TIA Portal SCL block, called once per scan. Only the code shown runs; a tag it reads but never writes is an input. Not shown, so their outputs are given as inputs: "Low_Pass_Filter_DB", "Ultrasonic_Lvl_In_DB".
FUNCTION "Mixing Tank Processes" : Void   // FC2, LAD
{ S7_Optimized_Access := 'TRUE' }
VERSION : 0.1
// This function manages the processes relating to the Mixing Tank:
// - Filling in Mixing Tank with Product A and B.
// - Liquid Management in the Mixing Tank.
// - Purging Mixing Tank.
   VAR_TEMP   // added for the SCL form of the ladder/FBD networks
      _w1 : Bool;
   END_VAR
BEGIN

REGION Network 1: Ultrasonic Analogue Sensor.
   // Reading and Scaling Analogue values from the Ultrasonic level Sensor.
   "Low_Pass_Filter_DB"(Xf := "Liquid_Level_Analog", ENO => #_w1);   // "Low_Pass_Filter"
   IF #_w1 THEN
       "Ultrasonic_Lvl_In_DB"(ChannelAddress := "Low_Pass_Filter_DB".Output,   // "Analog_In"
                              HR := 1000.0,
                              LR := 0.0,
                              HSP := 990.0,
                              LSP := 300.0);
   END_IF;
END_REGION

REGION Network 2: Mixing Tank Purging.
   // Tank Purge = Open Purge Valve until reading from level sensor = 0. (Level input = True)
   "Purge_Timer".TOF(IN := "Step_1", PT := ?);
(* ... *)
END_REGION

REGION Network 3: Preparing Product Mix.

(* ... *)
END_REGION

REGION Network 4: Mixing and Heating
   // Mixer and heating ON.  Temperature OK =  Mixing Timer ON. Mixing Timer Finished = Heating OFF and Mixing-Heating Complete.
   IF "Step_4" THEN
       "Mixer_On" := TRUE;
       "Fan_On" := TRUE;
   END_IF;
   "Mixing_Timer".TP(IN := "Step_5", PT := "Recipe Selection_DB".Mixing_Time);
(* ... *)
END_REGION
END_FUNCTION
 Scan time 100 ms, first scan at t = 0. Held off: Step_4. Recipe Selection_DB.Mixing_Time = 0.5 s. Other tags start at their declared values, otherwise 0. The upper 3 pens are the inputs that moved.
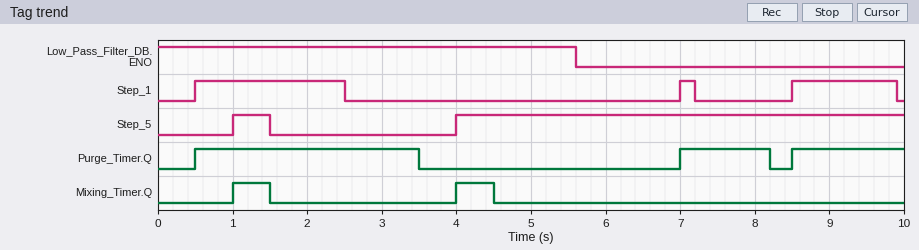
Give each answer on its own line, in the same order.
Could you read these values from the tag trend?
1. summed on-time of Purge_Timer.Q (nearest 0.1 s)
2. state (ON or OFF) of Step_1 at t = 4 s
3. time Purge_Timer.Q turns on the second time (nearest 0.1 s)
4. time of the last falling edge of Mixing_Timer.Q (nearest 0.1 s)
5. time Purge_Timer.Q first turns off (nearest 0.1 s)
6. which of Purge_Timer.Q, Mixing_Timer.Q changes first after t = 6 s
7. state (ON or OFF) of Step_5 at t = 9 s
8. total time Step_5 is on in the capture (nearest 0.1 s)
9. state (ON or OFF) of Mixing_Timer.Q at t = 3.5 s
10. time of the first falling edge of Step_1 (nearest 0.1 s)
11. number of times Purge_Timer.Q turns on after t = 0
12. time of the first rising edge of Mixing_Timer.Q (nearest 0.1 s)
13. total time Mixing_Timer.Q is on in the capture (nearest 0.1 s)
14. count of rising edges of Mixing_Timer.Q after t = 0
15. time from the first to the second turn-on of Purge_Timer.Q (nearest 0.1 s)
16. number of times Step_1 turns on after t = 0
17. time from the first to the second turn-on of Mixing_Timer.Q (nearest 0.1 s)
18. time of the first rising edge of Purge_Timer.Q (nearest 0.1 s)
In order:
5.7 s
OFF
7.0 s
4.5 s
3.5 s
Purge_Timer.Q
ON
6.5 s
OFF
2.5 s
3
1.0 s
1.0 s
2
6.5 s
3
3.0 s
0.5 s
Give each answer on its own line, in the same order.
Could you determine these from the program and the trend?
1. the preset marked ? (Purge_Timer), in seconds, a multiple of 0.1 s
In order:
1.0 s
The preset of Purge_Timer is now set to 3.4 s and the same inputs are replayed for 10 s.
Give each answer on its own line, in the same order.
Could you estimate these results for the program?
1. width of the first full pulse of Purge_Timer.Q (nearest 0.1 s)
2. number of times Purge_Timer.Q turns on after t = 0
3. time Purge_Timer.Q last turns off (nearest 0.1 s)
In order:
5.4 s
2
5.9 s
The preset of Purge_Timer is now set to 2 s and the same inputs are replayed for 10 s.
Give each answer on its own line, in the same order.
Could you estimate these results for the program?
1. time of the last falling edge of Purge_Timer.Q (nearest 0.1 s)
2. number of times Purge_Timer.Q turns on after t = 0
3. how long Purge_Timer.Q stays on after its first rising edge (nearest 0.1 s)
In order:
4.5 s
2
4.0 s
